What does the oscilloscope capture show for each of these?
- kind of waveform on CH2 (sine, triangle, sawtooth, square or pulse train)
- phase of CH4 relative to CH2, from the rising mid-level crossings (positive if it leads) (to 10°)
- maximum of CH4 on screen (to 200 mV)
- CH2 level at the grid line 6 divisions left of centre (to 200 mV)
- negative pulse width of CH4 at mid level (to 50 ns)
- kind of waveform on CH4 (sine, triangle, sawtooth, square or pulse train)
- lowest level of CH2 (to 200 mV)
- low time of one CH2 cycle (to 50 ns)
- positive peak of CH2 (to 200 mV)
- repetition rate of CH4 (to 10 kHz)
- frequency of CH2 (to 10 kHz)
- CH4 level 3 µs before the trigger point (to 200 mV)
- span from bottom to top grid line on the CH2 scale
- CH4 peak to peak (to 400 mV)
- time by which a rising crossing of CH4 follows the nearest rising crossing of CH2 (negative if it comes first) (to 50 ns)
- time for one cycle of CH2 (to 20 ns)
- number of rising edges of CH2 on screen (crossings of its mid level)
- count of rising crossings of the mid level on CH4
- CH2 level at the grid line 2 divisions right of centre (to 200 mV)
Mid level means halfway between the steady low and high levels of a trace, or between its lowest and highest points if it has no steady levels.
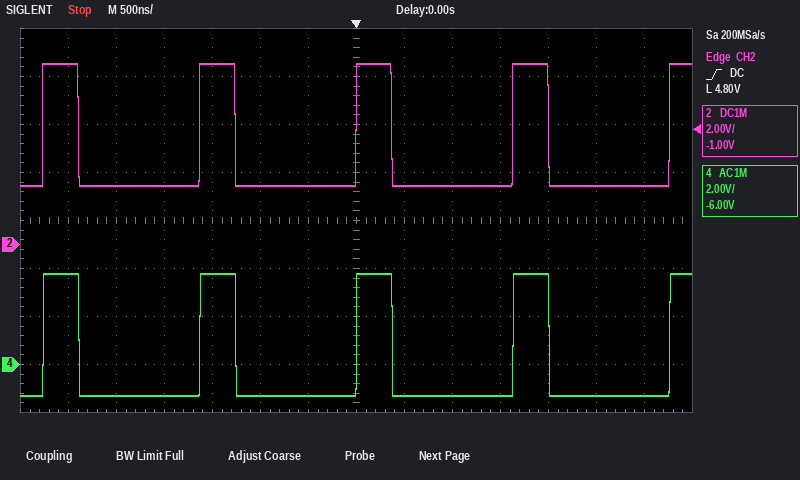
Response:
pulse train
0°
3.8 V
7.6 V
1.25 µs
pulse train
2.4 V
1.25 µs
7.6 V
610 kHz
610 kHz
3.8 V
16 V
5.2 V
0 ns
1.64 µs
5
5
2.4 V
